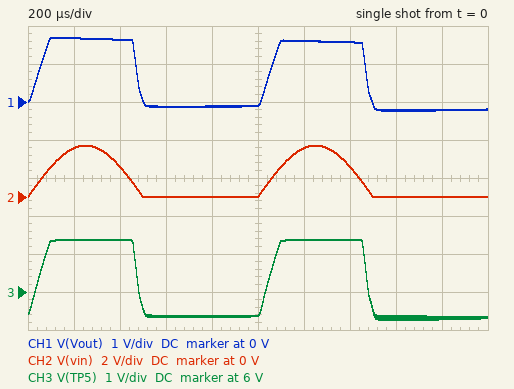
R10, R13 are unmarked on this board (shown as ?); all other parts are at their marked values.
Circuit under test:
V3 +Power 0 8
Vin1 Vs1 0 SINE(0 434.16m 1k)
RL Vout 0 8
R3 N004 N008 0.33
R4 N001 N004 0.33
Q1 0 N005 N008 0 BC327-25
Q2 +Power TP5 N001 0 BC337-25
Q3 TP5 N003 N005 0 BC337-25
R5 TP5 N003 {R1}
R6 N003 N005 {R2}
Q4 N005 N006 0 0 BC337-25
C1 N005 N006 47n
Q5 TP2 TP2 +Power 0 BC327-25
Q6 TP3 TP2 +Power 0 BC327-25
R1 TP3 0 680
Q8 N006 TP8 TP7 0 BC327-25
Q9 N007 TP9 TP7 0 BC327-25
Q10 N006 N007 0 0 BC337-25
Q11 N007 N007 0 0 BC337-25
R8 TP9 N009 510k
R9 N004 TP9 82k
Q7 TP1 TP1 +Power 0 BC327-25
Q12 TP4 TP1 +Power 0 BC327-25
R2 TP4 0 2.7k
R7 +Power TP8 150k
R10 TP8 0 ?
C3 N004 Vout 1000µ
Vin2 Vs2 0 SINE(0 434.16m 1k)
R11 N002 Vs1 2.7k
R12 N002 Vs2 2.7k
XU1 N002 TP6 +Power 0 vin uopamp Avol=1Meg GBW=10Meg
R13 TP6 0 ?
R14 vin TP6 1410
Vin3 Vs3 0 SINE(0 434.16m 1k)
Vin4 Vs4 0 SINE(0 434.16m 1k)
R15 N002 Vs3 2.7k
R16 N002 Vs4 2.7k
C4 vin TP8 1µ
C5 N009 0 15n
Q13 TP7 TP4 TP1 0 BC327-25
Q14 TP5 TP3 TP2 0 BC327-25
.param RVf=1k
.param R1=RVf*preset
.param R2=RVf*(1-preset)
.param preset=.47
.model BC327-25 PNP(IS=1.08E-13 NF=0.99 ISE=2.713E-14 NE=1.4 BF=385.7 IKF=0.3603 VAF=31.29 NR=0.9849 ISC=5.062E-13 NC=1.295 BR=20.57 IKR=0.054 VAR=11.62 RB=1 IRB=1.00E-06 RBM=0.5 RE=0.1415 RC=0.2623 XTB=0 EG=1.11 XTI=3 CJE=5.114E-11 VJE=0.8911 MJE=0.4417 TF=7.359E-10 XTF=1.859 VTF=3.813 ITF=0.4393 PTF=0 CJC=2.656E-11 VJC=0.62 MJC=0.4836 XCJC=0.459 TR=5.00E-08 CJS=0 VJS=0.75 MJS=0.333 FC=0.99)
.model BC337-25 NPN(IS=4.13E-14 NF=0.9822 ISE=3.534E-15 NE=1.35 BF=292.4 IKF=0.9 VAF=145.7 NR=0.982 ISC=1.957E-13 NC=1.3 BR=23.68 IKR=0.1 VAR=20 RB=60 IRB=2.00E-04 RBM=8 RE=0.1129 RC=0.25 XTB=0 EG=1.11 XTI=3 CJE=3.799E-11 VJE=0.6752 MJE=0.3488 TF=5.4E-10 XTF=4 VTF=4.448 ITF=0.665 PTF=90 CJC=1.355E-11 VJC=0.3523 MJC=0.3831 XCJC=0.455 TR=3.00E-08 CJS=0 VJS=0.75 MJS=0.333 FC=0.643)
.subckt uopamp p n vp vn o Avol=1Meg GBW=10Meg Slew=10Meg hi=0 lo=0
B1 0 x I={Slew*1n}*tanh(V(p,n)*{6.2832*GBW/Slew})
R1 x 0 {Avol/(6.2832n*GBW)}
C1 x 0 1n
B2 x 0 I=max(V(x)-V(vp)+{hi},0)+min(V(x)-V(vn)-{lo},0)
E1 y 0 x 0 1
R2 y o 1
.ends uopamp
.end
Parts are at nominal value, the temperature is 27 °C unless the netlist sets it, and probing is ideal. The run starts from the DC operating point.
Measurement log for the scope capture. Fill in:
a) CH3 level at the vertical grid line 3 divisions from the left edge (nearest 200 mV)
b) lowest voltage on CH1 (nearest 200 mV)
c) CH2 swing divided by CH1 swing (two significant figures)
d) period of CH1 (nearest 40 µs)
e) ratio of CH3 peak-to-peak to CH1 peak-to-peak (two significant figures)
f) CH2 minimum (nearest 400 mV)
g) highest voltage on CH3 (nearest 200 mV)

5.4 V
-200 mV
1.4
1.00 ms
1.1
0 V
7.4 V
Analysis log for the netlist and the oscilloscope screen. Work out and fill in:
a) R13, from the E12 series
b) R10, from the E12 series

270 Ω
220 kΩ
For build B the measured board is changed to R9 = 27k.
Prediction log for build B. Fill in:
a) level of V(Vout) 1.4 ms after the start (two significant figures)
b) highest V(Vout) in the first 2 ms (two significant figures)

1.4 V
1.5 V
